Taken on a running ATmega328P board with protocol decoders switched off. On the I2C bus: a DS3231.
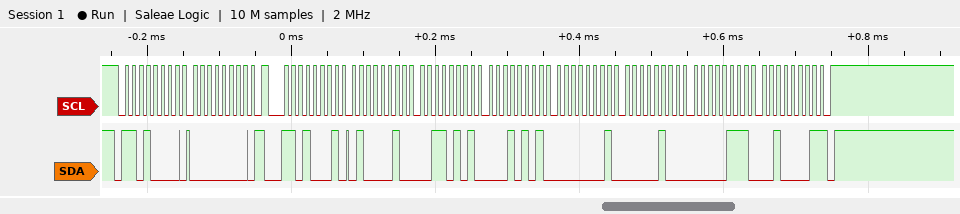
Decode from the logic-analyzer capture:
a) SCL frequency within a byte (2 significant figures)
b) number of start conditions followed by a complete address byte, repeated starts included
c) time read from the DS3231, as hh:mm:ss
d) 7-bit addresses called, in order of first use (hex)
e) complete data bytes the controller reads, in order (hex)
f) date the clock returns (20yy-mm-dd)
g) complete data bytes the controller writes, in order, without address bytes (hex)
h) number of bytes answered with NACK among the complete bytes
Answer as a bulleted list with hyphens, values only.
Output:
- 100 kHz
- 2
- 15:35:42
- 0x68
- 42 35 15 01 04 07 21
- 2021-07-04
- 00
- 1
